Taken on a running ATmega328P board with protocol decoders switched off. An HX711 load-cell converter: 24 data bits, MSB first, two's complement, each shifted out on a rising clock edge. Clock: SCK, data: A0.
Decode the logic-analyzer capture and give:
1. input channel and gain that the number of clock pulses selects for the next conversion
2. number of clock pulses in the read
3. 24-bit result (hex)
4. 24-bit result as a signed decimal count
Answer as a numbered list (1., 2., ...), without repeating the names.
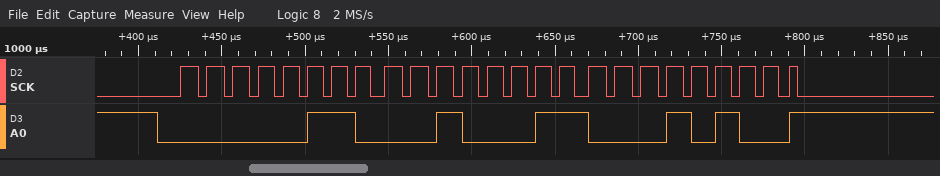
1. channel A, gain 128
2. 25
3. 0x062314
4. 402196
